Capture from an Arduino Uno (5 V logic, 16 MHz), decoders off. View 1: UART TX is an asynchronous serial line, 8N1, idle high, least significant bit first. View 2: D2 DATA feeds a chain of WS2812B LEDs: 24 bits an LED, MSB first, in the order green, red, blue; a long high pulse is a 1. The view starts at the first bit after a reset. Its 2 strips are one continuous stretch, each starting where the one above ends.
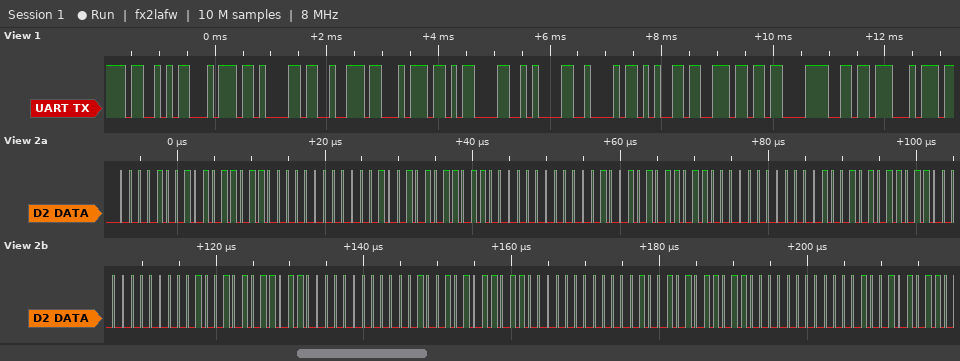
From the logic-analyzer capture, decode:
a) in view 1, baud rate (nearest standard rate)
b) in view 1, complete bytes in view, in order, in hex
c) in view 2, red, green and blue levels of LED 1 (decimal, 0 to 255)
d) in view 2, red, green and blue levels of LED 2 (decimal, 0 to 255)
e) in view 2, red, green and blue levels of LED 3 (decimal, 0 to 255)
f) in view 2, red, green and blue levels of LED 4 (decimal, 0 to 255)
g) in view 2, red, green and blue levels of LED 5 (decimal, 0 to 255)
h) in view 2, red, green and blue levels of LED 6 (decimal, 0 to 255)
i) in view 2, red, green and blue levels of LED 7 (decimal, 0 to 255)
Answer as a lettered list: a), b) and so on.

a) 9600 baud
b) 53 74 61 72 74 0D 0A 42 65 6E C3 B6 74
c) 91, 9, 0
d) 91, 9, 0
e) 91, 9, 0
f) 91, 9, 0
g) 91, 9, 0
h) 91, 9, 0
i) 91, 9, 0
